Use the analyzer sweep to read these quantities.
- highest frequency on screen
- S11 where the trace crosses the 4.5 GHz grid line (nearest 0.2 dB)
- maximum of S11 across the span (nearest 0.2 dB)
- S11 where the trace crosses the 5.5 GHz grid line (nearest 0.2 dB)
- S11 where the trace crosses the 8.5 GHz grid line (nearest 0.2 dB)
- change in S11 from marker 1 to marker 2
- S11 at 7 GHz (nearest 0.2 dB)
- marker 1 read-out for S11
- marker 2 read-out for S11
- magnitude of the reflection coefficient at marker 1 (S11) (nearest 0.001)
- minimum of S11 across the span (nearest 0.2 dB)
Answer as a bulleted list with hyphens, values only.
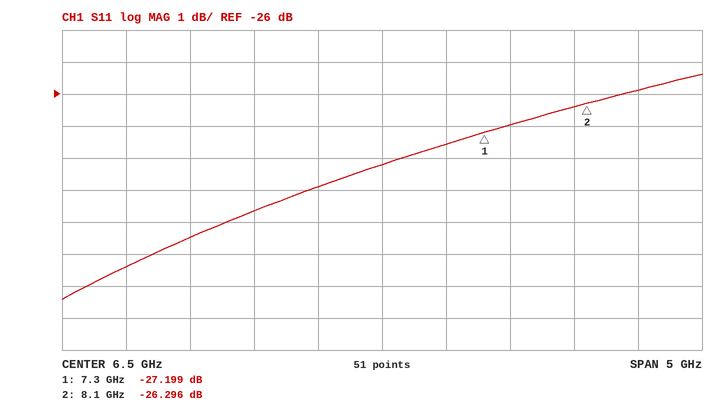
- 9 GHz
- -31.4 dB
- -25.4 dB
- -29.6 dB
- -25.8 dB
- 0.903 dB
- -27.6 dB
- -27.199 dB
- -26.296 dB
- 0.044
- -32.4 dB
